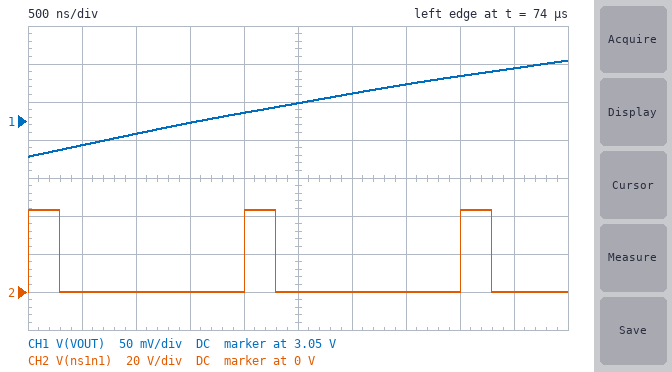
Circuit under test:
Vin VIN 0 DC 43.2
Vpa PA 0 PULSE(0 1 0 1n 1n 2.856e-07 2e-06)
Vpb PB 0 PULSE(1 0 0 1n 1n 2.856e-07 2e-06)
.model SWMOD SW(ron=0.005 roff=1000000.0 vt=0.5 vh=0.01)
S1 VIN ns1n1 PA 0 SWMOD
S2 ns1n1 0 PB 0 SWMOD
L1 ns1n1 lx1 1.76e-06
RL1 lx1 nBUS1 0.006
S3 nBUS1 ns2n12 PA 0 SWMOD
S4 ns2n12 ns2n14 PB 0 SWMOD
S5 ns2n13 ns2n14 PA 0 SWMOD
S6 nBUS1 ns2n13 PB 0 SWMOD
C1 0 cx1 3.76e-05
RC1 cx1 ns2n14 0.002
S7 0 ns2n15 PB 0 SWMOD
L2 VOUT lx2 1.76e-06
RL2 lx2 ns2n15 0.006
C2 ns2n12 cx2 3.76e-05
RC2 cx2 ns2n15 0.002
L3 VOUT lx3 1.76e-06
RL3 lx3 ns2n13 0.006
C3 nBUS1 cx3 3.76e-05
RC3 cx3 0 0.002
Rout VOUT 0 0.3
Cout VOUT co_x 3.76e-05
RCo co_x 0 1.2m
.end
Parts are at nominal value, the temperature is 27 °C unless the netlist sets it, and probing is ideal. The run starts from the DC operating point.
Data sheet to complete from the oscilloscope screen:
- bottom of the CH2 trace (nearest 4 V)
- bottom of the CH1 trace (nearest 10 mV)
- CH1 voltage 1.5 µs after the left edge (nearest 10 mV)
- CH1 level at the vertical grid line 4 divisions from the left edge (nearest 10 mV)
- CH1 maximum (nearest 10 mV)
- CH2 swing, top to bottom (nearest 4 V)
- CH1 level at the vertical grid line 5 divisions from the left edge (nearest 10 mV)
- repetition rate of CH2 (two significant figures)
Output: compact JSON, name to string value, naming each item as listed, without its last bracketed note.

{"bottom of the CH2 trace": "0 V", "bottom of the CH1 trace": "3.00 V", "CH1 voltage 1.5 µs after the left edge": "3.05 V", "CH1 level at the vertical grid line 4 divisions from the left edge": "3.06 V", "CH1 maximum": "3.13 V", "CH2 swing, top to bottom": "44 V", "CH1 level at the vertical grid line 5 divisions from the left edge": "3.07 V", "repetition rate of CH2": "500 kHz"}
